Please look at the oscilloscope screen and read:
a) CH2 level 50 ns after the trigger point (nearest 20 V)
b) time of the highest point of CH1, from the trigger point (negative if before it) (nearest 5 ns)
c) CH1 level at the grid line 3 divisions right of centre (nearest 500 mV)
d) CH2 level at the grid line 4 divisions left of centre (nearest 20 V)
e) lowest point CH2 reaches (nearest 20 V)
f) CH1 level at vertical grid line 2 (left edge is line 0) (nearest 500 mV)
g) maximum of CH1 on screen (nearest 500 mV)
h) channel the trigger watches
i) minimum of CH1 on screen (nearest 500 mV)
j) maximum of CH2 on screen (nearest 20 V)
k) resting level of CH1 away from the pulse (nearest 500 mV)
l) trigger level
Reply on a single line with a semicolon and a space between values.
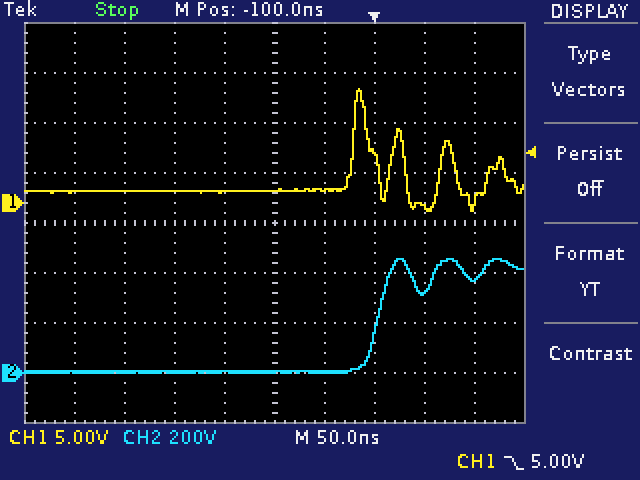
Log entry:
320 V; -15 ns; -500 mV; 0 V; 0 V; 1.0 V; 11.5 V; CH1; -1.0 V; 460 V; 1.0 V; 5.00 V
